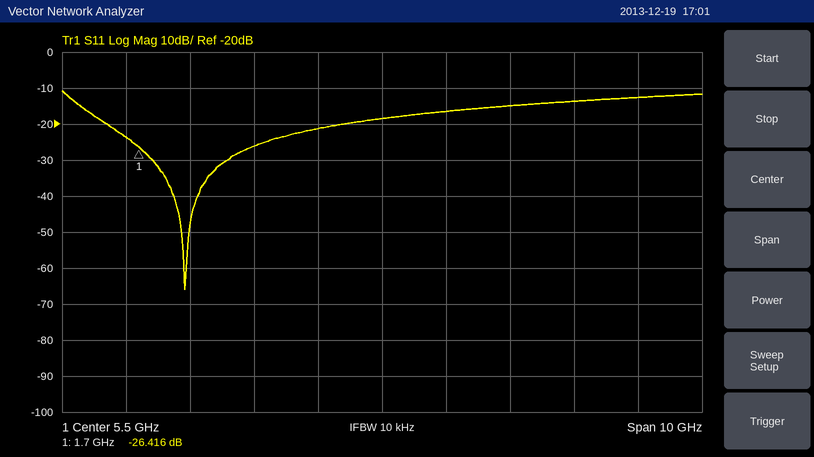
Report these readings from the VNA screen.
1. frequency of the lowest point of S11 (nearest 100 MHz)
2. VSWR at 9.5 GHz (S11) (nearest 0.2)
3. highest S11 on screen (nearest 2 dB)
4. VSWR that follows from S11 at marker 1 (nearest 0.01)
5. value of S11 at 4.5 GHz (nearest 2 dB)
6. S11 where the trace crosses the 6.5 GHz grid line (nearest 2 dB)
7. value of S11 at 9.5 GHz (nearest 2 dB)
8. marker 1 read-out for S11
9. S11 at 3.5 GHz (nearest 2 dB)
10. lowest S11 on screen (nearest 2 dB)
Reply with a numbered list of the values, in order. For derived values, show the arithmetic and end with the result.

1. 2.4 GHz
2. |Γ| = 10^(-12/20) = 0.2512; VSWR = (1 + 0.2512)/(1 − 0.2512) ≈ 1.67, so 1.6 to the nearest 0.2
3. -10 dB
4. (1 + 0.0478)/(1 − 0.0478) ≈ 1.10
5. -22 dB
6. -16 dB
7. -12 dB
8. -26.416 dB
9. -26 dB
10. -66 dB
